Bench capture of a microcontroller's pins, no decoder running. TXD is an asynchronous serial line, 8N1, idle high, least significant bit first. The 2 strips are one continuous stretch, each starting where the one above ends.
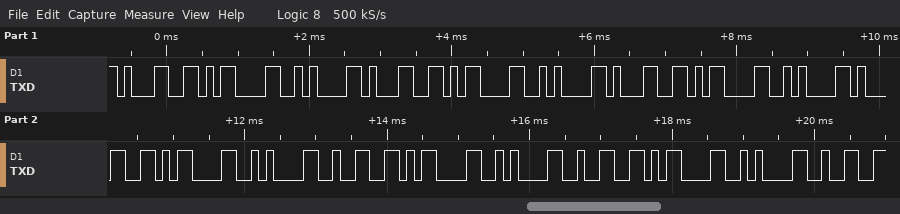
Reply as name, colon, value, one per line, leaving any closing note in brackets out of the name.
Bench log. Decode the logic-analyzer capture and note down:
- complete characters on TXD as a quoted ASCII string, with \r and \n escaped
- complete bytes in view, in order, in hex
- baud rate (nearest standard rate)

complete characters on TXD as a quoted ASCII string, with \r and \n escaped: "1\r\n1\r\n1\r\n1\r\n2\r\n2\r\n2"
complete bytes in view, in order, in hex: 31 0D 0A 31 0D 0A 31 0D 0A 31 0D 0A 32 0D 0A 32 0D 0A 32
baud rate: 9600 baud
